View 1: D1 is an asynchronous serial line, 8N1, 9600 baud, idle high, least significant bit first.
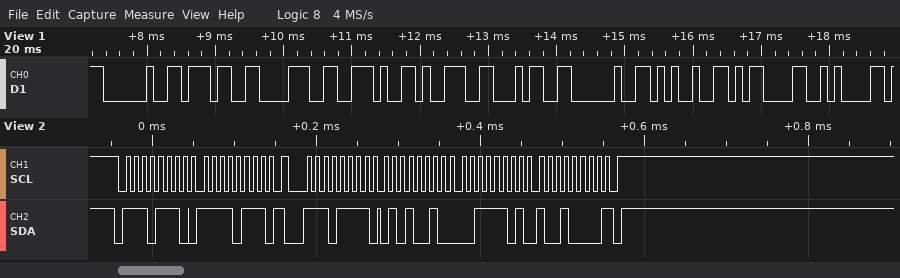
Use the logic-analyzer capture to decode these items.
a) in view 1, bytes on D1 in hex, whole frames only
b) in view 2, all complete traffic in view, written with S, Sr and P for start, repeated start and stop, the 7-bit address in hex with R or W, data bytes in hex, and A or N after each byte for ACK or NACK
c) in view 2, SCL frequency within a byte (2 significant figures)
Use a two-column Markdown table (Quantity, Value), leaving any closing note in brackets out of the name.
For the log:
| Quantity | Value |
|---|---|
| in view 1, bytes on D1 in hex, whole frames only | 0x20 0x37 0x38 0x2E 0x39 0x34 0x20 0x25 0x0D 0x0A |
| in view 2, all complete traffic in view, written with S, Sr and P for start, repeated start and stop, the 7-bit address in hex with R or W, data bytes in hex, and A or N after each byte for ACK or NACK | S 77W A F7 A Sr 77R A 52 A 3D A 90 N P |
| in view 2, SCL frequency within a byte | 100 kHz |
